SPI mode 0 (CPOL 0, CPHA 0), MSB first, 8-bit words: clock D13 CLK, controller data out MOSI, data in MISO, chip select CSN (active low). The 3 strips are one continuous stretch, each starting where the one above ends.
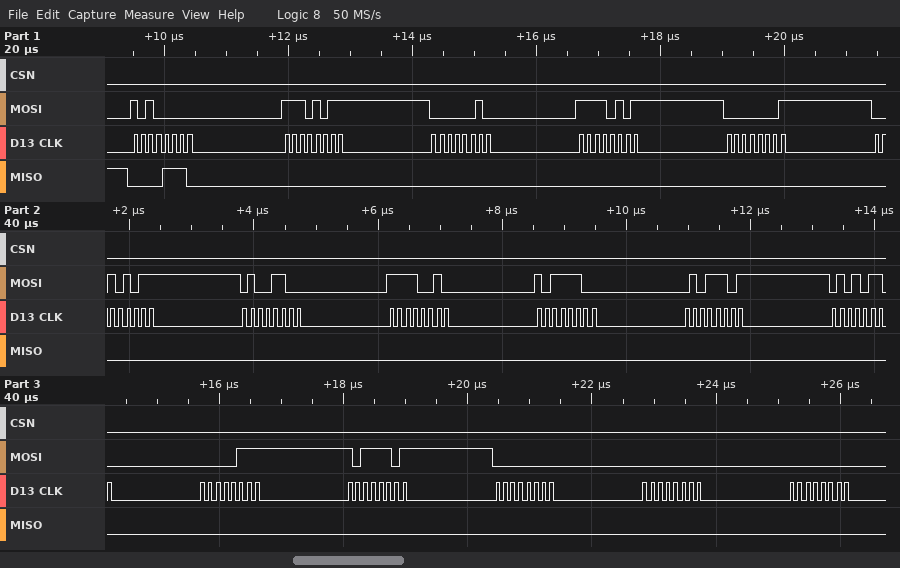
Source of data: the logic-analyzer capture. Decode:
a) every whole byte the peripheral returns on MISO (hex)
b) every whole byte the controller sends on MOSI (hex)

0E 00 00 00 00 00 00 00 00 00 00 00 00 00 00 00
A0 EB 02 F5 01 2B 4C F2 BC 5D 56 07 BD 00 00 00
